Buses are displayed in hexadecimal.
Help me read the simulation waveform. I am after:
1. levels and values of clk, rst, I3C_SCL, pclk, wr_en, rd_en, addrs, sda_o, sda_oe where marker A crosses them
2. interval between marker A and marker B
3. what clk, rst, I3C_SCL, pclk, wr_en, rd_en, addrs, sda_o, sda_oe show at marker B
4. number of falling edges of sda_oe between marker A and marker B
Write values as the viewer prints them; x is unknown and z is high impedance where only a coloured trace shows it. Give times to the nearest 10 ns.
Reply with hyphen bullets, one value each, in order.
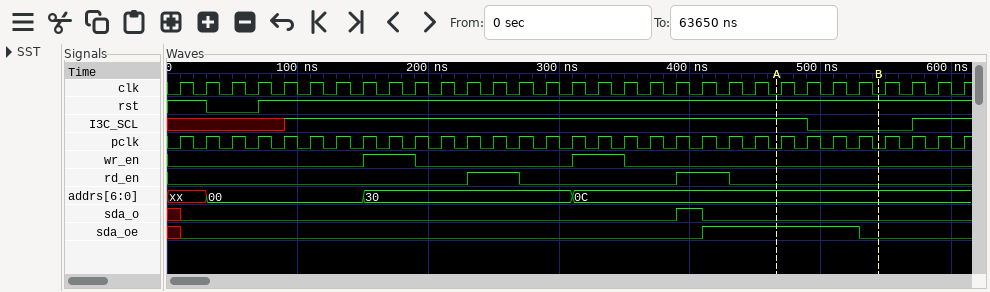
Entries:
- clk=0, rst=1, I3C_SCL=1, pclk=0, wr_en=0, rd_en=0, addrs=0C, sda_o=0, sda_oe=1
- 80 ns
- clk=0, rst=1, I3C_SCL=0, pclk=0, wr_en=0, rd_en=0, addrs=0C, sda_o=0, sda_oe=0
- 1
